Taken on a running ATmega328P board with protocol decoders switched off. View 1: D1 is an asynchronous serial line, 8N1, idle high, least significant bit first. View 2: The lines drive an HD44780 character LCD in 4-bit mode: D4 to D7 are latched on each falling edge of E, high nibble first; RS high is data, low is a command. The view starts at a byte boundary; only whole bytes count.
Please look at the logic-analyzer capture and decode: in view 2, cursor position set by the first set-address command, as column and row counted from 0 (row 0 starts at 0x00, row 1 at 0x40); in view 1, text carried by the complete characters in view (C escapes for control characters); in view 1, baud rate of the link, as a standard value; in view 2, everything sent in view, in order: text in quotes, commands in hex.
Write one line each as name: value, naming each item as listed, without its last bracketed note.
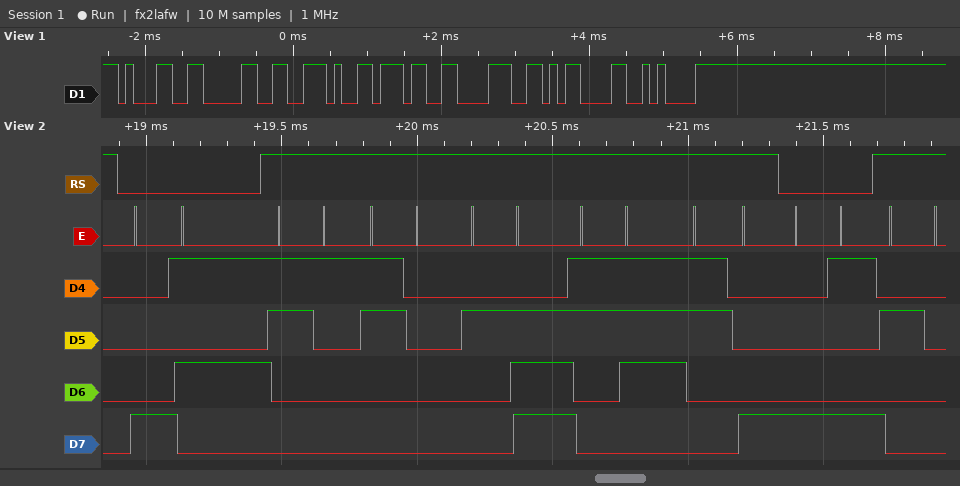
in view 2, cursor position set by the first set-address command, as column and row counted from 0: column 5, row 0
in view 1, text carried by the complete characters in view: "10.78\r\n"
in view 1, baud rate of the link, as a standard value: 9600 baud
in view 2, everything sent in view, in order: text in quotes, commands in hex: 0x85 "10.78" 0x89 " "
